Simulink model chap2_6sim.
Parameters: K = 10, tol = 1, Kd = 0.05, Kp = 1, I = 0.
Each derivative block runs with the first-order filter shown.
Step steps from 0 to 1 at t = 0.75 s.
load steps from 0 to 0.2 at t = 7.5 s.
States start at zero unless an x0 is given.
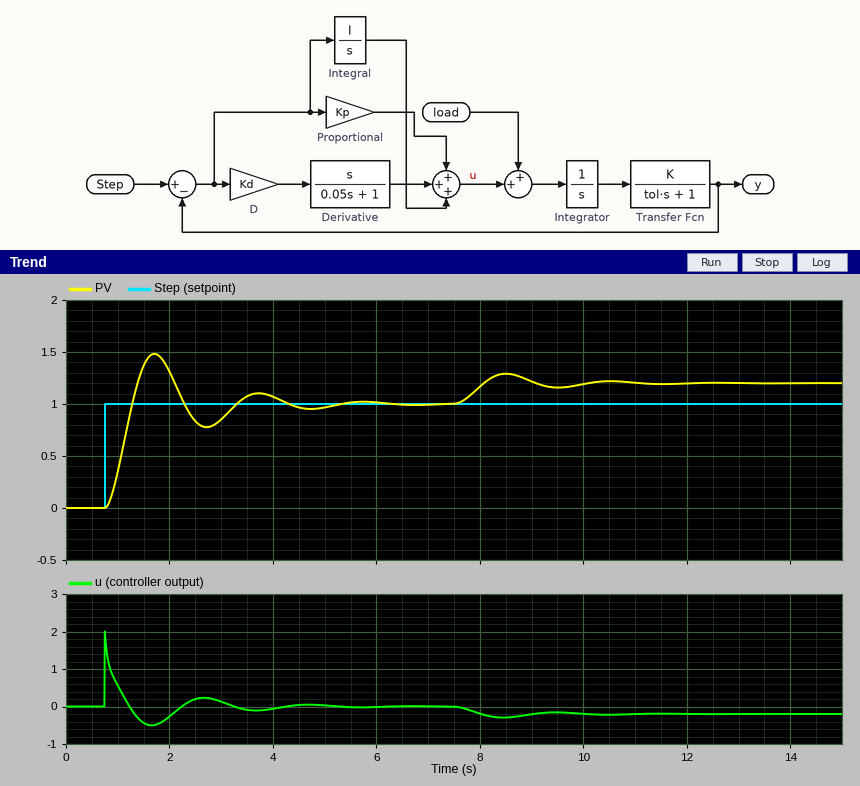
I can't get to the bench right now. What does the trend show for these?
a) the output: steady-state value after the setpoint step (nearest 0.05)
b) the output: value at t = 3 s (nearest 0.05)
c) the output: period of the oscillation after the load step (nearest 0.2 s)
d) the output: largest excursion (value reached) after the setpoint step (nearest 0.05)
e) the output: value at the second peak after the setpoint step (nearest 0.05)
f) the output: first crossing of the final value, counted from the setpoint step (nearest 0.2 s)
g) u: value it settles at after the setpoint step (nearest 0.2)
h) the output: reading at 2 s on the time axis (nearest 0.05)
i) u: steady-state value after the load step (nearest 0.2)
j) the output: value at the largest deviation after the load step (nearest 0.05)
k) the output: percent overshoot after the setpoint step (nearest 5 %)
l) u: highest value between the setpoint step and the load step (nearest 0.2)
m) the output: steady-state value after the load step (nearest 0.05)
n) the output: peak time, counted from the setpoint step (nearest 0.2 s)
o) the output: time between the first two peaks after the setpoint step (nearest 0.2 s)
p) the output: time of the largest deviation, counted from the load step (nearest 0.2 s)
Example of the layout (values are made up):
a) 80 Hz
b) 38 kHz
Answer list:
a) 1.00
b) 0.85
c) 2.0 s
d) 1.50
e) 1.10
f) 0.6 s
g) 0.0
h) 1.30
i) -0.2
j) 1.30
k) 50 %
l) 2.0
m) 1.20
n) 1.0 s
o) 2.0 s
p) 1.0 s
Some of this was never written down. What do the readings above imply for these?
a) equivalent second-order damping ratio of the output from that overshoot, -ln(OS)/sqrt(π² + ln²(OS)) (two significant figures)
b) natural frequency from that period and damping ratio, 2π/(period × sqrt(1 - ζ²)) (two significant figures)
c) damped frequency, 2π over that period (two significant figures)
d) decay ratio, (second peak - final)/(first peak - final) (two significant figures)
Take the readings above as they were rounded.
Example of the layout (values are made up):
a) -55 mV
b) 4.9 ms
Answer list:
a) 0.22
b) 3.2 rad/s
c) 3.1 rad/s
d) 0.20
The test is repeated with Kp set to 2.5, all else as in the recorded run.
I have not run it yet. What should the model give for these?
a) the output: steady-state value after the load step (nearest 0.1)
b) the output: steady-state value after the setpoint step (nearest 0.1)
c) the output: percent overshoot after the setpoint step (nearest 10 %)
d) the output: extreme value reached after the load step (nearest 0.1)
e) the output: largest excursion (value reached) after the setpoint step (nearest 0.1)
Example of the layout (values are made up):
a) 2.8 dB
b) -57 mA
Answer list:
a) 1.1
b) 1.0
c) 60 %
d) 1.1
e) 1.6
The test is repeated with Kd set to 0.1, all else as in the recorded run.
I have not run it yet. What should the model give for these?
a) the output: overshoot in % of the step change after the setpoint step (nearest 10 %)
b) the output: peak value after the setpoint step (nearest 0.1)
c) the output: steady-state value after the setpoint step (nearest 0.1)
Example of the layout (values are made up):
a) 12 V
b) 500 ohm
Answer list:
a) 40 %
b) 1.4
c) 1.0
